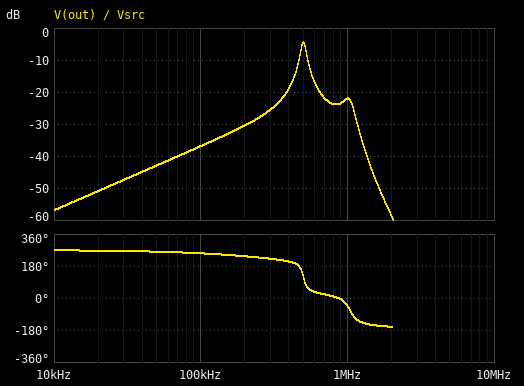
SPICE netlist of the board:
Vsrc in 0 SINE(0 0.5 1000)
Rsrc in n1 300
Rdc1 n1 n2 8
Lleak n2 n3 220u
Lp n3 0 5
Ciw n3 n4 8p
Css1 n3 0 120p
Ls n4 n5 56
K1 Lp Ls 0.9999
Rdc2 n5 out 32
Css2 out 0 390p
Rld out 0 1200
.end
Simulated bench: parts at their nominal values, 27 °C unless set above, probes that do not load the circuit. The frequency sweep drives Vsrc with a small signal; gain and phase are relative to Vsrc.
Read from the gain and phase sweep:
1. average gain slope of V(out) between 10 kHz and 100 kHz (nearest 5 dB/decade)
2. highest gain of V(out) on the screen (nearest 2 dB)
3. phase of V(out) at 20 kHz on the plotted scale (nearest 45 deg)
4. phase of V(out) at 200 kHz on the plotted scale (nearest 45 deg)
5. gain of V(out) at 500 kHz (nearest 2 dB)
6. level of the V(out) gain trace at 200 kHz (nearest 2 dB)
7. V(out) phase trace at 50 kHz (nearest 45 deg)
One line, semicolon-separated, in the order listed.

20 dB/decade; -4 dB; 270 deg; 225 deg; -4 dB; -30 dB; 270 deg
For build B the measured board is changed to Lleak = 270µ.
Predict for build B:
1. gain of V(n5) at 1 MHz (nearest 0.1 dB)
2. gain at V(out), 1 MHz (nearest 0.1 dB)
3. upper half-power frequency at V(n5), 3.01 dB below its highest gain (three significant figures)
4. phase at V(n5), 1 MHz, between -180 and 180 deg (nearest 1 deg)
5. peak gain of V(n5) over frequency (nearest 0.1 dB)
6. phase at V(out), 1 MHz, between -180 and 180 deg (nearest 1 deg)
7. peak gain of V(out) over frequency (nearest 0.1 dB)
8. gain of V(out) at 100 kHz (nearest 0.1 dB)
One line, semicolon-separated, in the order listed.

-21.4 dB; -21.7 dB; 515 kHz; -92 deg; -4.4 dB; -96 deg; -4.6 dB; -36.9 dB
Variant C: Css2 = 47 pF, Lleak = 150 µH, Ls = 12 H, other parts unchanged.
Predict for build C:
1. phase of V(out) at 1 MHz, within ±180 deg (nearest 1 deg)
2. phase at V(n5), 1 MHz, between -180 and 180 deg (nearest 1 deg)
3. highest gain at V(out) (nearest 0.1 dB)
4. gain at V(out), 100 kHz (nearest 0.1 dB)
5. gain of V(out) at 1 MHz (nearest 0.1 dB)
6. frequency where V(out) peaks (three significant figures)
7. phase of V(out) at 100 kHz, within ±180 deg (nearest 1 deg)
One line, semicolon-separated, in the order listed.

-169 deg; -168 deg; -0.3 dB; -49.5 dB; -9.6 dB; 1.17 MHz; -94 deg
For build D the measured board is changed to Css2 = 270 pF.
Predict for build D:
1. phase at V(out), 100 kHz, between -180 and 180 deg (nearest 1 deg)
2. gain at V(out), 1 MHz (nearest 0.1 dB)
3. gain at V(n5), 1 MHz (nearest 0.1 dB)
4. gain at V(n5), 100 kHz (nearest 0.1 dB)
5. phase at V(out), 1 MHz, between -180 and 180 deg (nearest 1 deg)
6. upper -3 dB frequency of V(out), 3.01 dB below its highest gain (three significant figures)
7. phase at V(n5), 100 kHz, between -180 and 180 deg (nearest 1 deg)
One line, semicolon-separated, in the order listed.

-104 deg; -19.2 dB; -19.0 dB; -36.5 dB; -35 deg; 525 kHz; -103 deg
